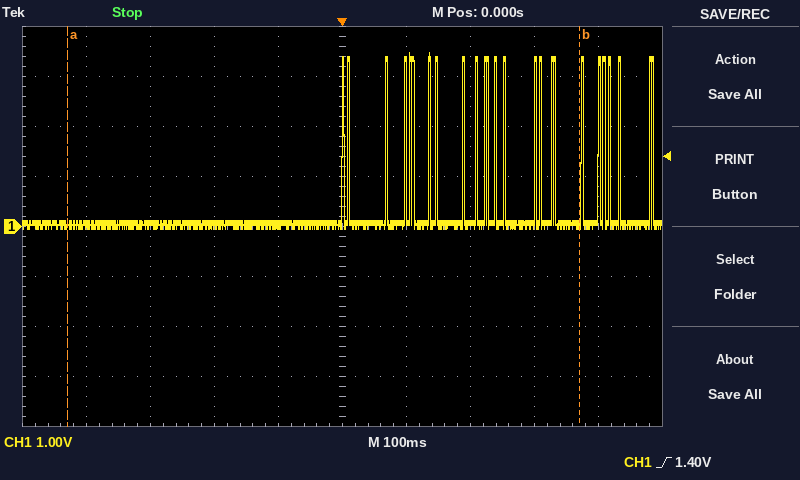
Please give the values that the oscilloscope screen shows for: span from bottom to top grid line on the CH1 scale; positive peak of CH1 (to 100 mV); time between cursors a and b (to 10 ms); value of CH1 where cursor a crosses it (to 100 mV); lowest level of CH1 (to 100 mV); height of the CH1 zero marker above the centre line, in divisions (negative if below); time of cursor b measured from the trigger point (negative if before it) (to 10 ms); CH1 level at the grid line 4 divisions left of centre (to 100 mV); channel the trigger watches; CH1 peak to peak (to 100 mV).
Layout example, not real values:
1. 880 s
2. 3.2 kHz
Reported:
1. 8 V
2. 3.5 V
3. 800 ms
4. 0.0 V
5. 0.0 V
6. 0.0 div
7. +370 ms
8. 0.0 V
9. CH1
10. 3.5 V
